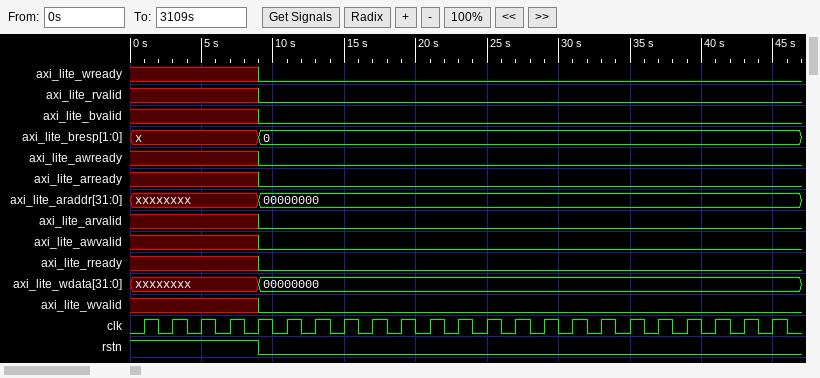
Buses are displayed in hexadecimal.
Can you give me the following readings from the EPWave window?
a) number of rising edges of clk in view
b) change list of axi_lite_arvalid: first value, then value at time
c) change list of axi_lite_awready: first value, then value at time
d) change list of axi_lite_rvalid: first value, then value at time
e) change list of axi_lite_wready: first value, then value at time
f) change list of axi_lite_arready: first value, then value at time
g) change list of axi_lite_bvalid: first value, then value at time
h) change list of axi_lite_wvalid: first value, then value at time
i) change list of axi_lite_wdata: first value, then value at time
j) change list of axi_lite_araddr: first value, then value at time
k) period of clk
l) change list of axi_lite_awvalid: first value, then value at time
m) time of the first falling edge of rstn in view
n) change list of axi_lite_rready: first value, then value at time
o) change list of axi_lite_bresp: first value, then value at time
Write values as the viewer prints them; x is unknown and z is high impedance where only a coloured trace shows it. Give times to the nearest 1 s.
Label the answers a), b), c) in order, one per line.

a) 23
b) x, 0 at 9 s
c) x, 0 at 9 s
d) x, 0 at 9 s
e) x, 0 at 9 s
f) x, 0 at 9 s
g) x, 0 at 9 s
h) x, 0 at 9 s
i) xxxxxxxx, 00000000 at 9 s
j) xxxxxxxx, 00000000 at 9 s
k) 2 s
l) x, 0 at 9 s
m) 9 s
n) x, 0 at 9 s
o) x, 0 at 9 s
